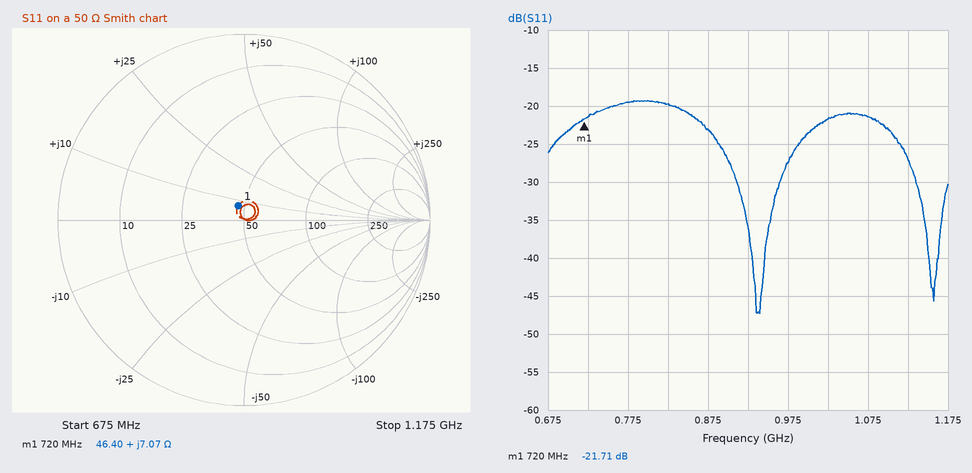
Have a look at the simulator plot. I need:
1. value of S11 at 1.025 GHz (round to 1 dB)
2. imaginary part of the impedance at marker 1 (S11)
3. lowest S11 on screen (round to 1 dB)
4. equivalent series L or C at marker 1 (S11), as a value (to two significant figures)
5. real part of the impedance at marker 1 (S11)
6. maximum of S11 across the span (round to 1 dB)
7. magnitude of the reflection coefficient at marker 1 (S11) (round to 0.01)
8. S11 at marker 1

-22 dB
+7.07 Ω
-47 dB
1.6 nH
46.40 Ω
-19 dB
0.08
-21.71 dB
